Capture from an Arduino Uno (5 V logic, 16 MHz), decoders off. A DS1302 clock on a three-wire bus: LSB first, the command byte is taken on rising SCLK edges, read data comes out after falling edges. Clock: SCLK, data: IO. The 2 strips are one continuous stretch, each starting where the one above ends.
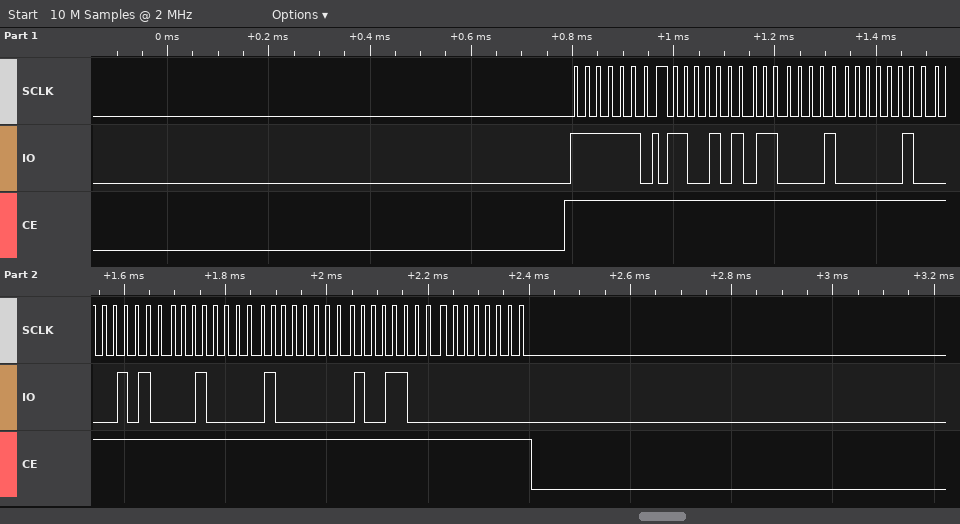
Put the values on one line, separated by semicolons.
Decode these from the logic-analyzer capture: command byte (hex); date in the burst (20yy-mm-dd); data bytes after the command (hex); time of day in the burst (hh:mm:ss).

0xBF; 2019-04-28; 53 43 20 28 04 01 19 00; 20:43:53
